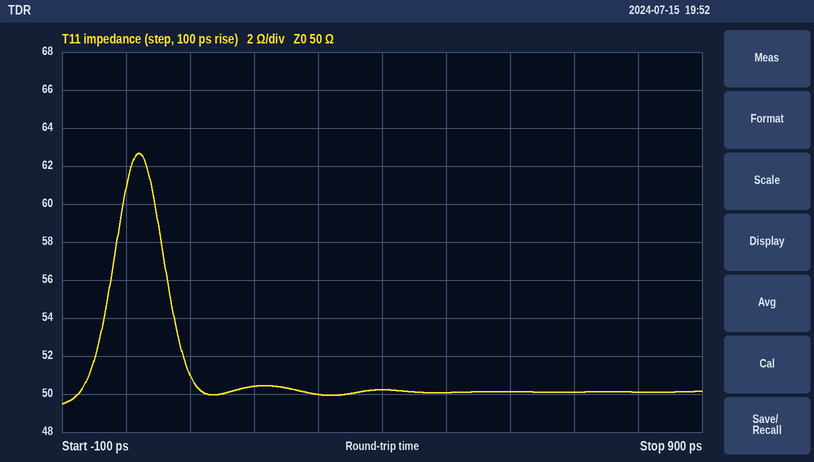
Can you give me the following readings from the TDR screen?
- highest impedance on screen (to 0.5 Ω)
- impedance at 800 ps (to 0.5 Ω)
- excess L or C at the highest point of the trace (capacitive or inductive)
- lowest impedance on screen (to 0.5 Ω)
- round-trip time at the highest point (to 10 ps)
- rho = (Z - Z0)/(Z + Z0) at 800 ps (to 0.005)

62.5 Ω
50.0 Ω
inductive
49.5 Ω
20 ps
0.000
